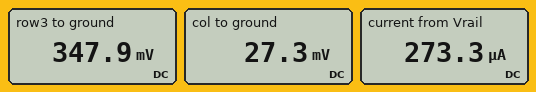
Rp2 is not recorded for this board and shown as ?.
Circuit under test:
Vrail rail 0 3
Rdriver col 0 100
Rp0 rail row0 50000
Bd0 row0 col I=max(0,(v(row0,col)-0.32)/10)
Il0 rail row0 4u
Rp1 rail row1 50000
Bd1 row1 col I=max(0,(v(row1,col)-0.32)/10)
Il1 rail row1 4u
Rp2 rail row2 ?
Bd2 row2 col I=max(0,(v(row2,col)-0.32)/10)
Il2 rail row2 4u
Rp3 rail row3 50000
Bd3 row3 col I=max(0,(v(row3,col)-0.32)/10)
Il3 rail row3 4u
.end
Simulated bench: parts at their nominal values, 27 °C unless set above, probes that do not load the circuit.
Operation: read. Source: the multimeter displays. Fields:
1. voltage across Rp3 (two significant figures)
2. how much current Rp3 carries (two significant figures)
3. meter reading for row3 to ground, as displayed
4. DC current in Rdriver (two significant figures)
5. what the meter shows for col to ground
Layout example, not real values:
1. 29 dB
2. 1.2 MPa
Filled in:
1. 2.7 V
2. 53 µA
3. 347.9 mV
4. 270 µA
5. 27.3 mV
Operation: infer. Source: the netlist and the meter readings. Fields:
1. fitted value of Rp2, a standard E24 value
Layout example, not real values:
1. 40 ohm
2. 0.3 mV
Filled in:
1. 27 kΩ
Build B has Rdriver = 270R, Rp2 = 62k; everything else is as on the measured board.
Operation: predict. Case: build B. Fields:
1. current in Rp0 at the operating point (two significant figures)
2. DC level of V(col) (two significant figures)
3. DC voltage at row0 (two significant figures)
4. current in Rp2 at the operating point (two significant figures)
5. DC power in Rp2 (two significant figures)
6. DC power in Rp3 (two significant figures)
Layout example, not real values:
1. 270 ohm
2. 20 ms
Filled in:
1. 52 µA
2. 58 mV
3. 380 mV
4. 42 µA
5. 110 µW
6. 140 µW
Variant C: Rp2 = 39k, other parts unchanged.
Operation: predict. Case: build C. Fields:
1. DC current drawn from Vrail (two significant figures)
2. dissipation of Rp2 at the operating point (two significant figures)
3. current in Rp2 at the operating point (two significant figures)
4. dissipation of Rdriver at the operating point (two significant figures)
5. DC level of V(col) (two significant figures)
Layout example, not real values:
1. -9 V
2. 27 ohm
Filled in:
1. 240 µA
2. 180 µW
3. 68 µA
4. 5.9 µW
5. 24 mV
